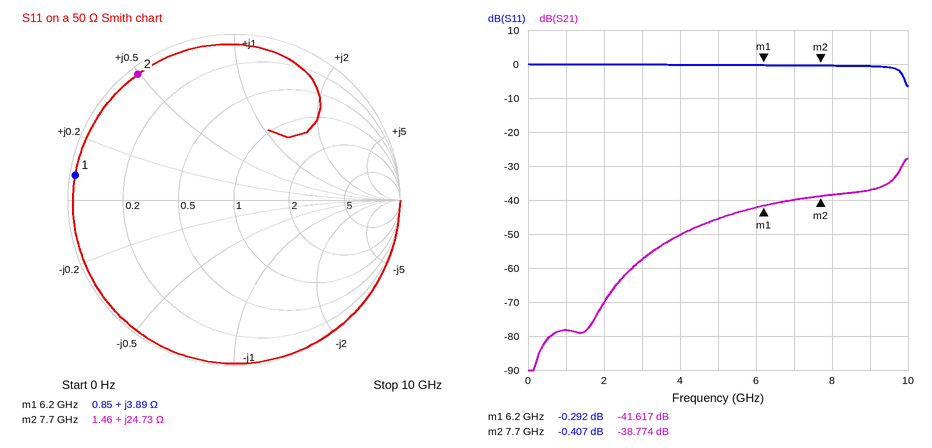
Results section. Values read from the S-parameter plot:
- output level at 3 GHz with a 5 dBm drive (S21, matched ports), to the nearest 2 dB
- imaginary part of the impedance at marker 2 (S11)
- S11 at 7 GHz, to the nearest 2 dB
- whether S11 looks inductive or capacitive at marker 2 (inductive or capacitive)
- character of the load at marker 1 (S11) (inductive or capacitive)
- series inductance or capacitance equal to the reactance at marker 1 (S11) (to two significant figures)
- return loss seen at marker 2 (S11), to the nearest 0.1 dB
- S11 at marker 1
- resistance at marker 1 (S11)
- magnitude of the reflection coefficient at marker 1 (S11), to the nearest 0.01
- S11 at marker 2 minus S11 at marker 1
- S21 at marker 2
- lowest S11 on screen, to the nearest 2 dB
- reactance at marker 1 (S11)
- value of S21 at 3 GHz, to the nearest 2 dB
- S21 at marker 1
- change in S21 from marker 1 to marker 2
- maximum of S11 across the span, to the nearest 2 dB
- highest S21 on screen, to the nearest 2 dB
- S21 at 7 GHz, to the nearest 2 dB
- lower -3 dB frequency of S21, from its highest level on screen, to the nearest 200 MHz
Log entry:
-52 dBm
+24.73 Ω
0 dB
inductive
inductive
100 pH
0.4 dB
-0.292 dB
0.85 Ω
0.97
-0.115 dB
-38.774 dB
-6 dB
+3.89 Ω
-58 dB
-41.617 dB
2.843 dB
0 dB
-28 dB
-40 dB
9.8 GHz
